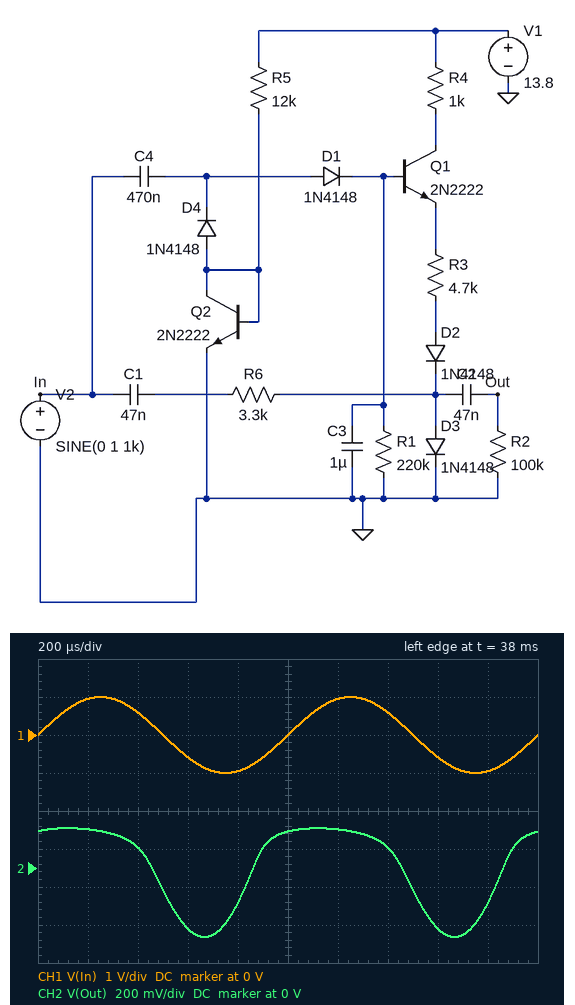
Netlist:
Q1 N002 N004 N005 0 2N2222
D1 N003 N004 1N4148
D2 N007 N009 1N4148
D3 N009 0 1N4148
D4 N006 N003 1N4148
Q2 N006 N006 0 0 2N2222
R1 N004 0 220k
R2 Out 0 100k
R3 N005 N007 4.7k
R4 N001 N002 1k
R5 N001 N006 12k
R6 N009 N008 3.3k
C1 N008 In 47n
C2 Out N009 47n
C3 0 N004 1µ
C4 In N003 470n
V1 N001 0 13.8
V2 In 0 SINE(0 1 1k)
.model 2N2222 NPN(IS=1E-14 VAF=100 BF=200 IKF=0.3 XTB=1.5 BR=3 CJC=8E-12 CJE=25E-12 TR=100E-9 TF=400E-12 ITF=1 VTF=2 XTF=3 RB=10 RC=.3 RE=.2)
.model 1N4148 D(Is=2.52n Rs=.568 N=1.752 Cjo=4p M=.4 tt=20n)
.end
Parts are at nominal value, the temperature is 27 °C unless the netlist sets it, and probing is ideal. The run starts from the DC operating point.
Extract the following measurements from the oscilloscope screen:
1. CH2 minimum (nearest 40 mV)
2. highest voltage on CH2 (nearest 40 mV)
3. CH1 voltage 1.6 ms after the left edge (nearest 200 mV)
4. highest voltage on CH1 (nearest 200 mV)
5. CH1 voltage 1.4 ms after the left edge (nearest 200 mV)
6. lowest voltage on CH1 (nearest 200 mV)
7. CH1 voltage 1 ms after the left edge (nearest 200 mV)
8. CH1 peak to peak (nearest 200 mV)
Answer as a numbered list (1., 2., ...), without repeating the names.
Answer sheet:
1. -360 mV
2. 200 mV
3. -600 mV
4. 1.0 V
5. 600 mV
6. -1.0 V
7. 0 V
8. 2.0 V
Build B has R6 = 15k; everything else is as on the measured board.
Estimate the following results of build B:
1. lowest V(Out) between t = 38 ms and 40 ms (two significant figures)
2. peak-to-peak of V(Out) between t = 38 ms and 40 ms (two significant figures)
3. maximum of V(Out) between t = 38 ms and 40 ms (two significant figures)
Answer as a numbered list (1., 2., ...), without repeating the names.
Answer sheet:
1. -81 mV
2. 130 mV
3. 52 mV
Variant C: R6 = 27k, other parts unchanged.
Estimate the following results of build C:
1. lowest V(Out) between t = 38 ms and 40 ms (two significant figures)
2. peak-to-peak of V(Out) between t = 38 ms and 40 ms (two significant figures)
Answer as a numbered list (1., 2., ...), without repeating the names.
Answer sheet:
1. -35 mV
2. 63 mV
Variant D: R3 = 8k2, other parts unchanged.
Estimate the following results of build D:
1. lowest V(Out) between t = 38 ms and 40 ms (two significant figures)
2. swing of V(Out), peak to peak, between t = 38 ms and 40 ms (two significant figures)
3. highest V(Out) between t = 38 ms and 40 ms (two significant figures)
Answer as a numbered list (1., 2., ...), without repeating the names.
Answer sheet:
1. -500 mV
2. 810 mV
3. 310 mV
